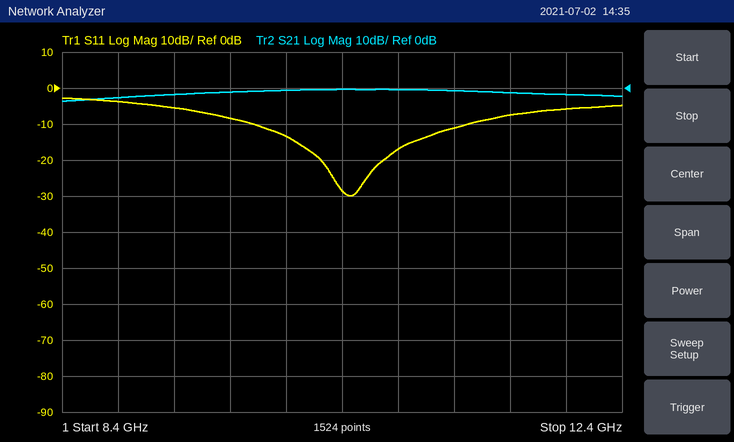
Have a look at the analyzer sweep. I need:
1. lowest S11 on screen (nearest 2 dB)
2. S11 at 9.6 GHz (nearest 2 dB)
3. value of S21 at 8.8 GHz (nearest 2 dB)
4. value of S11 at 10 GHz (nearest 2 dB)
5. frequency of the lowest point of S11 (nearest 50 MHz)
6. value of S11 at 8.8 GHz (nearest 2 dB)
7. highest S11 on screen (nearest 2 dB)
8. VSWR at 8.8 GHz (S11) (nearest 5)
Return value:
-30 dB
-8 dB
-2 dB
-14 dB
10.45 GHz
-4 dB
-2 dB
5
